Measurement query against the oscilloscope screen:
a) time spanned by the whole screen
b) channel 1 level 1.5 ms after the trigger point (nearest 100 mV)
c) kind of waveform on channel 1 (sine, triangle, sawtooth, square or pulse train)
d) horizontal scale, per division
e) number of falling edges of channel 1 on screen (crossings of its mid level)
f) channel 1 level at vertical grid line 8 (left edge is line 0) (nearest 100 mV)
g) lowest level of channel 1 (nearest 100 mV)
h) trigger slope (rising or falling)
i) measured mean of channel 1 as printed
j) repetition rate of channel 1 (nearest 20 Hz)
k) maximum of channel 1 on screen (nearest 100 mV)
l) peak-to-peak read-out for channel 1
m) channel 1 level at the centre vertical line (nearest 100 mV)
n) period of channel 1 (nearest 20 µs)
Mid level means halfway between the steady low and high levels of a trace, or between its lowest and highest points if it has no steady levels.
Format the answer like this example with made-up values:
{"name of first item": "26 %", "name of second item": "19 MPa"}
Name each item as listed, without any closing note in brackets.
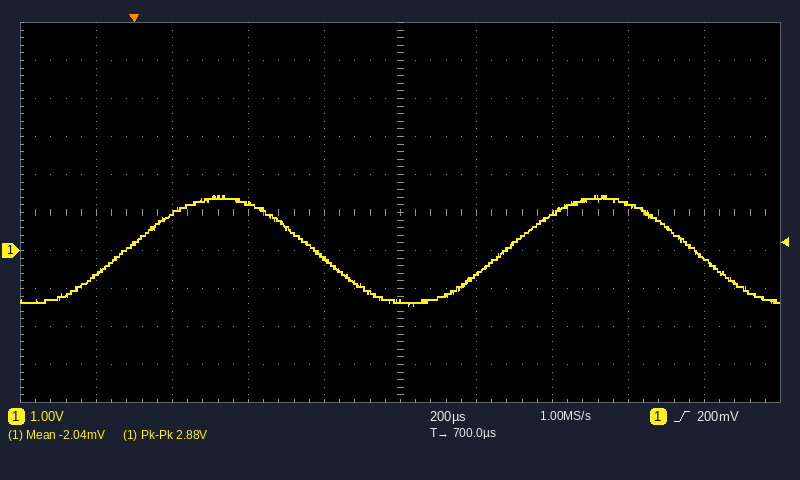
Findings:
{"time spanned by the whole screen": "2 ms", "channel 1 level 1.5 ms after the trigger point": "-200 mV", "kind of waveform on channel 1": "sine", "horizontal scale, per division": "200 µs", "number of falling edges of channel 1 on screen": "2", "channel 1 level at vertical grid line 8 (left edge is line 0)": "1.2 V", "lowest level of channel 1": "-1.4 V", "trigger slope": "rising", "measured mean of channel 1 as printed": "-2.04 mV", "repetition rate of channel 1": "1.00 kHz", "maximum of channel 1 on screen": "1.4 V", "peak-to-peak read-out for channel 1": "2.88 V", "channel 1 level at the centre vertical line": "-1.3 V", "period of channel 1": "1.00 ms"}
